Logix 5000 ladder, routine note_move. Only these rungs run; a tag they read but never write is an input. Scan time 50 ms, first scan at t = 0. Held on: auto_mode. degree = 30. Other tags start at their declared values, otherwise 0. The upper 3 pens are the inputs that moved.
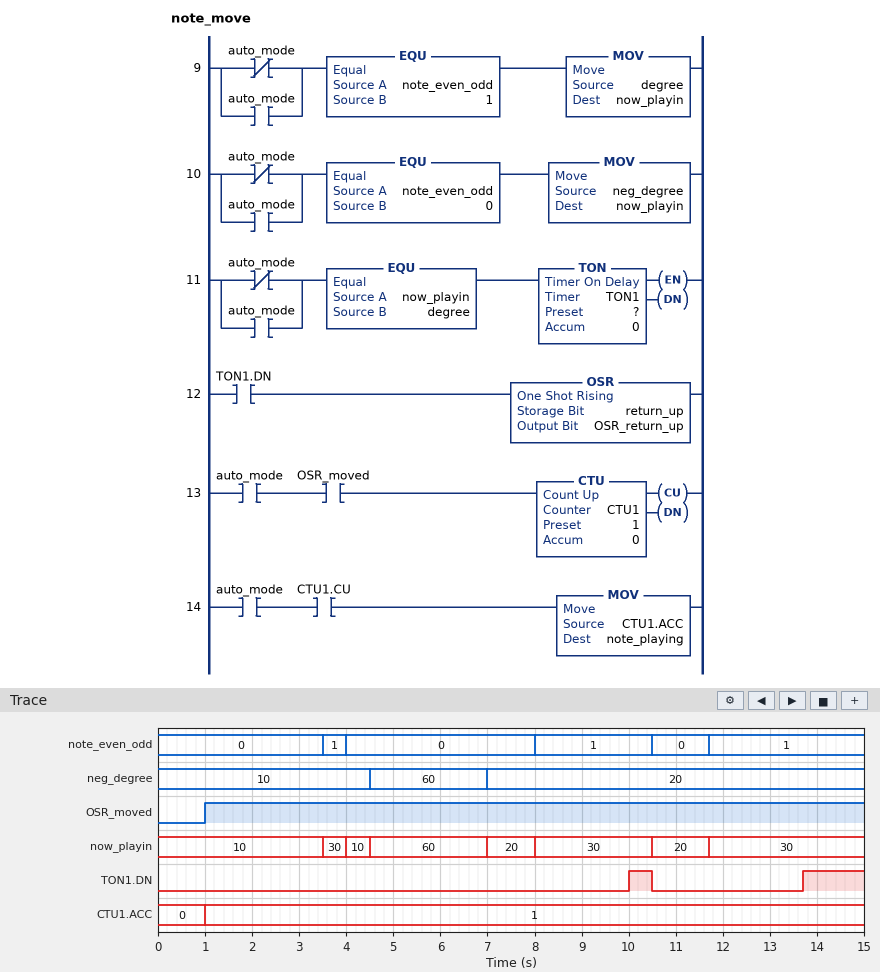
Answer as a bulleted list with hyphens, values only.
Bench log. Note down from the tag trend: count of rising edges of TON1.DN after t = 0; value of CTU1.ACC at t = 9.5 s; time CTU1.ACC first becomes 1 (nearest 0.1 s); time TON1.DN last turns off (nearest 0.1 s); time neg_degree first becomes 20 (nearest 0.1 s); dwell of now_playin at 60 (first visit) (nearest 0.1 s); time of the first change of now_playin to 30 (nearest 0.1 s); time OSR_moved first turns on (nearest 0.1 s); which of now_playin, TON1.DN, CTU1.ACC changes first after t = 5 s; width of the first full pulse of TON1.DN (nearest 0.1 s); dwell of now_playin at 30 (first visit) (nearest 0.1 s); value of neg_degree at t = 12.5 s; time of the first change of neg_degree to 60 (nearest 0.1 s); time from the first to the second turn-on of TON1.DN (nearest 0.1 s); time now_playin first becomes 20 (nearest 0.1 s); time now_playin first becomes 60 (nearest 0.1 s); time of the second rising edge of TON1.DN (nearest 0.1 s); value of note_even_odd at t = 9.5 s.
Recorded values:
- 2
- 1
- 1.0 s
- 10.5 s
- 7.0 s
- 2.5 s
- 3.5 s
- 1.0 s
- now_playin
- 0.5 s
- 0.5 s
- 20
- 4.5 s
- 3.7 s
- 7.0 s
- 4.5 s
- 13.7 s
- 1
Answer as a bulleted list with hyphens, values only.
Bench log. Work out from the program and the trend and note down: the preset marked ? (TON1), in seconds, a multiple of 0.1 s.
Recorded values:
- 2.0 s
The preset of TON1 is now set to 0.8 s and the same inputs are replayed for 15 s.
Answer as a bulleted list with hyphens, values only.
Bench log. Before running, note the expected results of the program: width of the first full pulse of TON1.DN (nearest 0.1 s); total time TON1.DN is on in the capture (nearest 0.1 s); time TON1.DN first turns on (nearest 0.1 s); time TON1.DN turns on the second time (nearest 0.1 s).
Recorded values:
- 1.7 s
- 4.2 s
- 8.8 s
- 12.5 s
